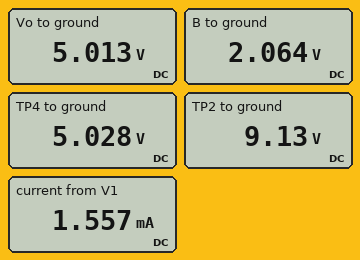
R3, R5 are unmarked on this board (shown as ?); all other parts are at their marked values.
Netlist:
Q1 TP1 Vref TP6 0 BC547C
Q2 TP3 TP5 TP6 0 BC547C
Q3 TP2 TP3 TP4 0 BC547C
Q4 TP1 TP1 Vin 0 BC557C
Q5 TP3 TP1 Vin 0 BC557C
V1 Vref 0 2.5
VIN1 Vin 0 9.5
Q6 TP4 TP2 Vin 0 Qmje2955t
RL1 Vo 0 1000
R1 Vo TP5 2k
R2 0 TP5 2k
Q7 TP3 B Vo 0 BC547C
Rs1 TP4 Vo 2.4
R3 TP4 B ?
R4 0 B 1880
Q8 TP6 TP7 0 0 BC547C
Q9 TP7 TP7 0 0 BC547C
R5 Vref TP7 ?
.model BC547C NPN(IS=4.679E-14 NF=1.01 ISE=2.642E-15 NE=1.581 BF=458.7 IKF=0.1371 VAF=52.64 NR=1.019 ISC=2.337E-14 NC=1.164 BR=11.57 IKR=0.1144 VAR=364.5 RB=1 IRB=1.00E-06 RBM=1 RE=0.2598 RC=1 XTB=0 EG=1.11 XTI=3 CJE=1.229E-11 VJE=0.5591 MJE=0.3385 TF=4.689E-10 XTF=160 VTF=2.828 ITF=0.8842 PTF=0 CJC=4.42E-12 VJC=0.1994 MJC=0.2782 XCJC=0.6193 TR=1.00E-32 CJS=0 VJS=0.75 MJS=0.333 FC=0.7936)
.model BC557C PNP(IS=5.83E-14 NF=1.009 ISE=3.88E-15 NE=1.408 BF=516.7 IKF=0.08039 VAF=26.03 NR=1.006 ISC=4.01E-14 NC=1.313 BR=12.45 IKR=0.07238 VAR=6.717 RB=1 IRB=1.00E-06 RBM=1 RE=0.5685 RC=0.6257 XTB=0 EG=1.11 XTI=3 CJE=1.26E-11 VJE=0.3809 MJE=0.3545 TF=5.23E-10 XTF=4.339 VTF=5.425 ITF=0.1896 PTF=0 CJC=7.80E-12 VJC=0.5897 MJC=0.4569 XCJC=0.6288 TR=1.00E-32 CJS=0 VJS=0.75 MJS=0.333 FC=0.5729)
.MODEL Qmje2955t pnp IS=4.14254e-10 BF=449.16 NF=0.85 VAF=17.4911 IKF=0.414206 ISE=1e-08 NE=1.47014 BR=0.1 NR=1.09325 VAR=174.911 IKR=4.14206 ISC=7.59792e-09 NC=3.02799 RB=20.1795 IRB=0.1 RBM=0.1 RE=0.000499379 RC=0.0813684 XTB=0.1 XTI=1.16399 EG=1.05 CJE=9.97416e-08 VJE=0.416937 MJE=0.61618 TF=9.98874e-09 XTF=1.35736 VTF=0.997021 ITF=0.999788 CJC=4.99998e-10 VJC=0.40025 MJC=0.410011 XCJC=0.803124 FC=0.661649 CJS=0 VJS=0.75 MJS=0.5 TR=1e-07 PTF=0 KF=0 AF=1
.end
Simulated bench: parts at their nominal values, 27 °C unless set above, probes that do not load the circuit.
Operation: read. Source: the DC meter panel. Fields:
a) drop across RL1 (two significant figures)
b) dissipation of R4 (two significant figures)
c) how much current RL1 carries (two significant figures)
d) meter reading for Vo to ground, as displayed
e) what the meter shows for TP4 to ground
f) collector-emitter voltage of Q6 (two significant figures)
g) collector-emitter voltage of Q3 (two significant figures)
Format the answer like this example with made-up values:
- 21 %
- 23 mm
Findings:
- 5.0 V
- 2.3 mW
- 5.0 mA
- 5.013 V
- 5.028 V
- -4.5 V
- 4.1 V
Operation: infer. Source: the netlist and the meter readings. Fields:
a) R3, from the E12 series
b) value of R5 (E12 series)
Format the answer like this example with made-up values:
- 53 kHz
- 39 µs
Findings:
- 2.7 kΩ
- 1.2 kΩ
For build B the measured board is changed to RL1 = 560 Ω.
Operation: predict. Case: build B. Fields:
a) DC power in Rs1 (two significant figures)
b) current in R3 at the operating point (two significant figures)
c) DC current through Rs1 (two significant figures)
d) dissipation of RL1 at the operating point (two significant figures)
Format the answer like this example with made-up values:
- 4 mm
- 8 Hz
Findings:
- 250 µW
- 1.1 mA
- 10 mA
- 45 mW
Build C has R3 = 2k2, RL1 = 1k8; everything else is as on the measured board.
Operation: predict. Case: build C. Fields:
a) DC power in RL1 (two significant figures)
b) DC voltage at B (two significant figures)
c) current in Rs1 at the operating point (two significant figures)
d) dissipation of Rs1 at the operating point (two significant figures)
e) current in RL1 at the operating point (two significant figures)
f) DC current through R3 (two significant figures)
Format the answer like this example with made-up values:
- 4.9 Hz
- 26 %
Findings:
- 14 mW
- 2.3 V
- 4.0 mA
- 39 µW
- 2.8 mA
- 1.2 mA
